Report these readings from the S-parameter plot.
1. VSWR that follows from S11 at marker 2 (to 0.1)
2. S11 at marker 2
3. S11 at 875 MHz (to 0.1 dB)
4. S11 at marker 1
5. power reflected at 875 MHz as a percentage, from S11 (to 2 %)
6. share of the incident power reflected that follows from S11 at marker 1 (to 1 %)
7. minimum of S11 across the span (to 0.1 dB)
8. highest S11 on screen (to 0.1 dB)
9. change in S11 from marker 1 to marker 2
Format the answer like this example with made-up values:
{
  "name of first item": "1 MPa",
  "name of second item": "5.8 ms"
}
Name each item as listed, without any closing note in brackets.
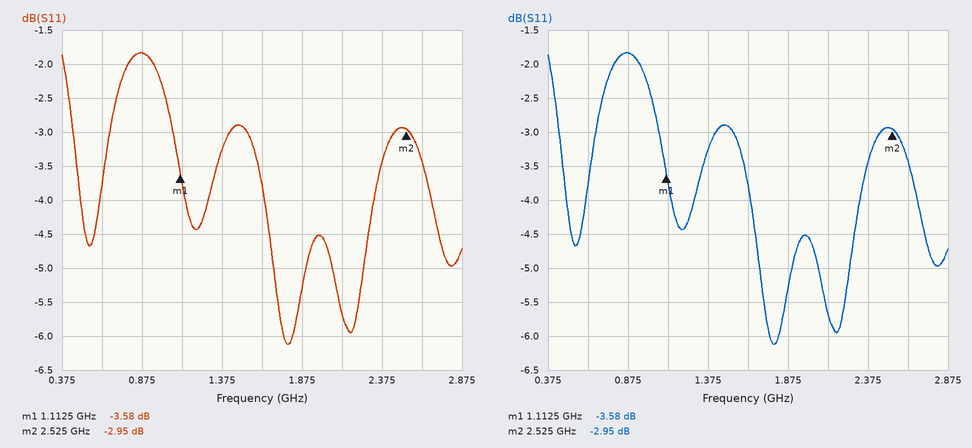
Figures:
{
  "VSWR that follows from S11 at marker 2": "5.9",
  "S11 at marker 2": "-2.95 dB",
  "S11 at 875 MHz": "-1.8 dB",
  "S11 at marker 1": "-3.58 dB",
  "power reflected at 875 MHz as a percentage, from S11": "66 %",
  "share of the incident power reflected that follows from S11 at marker 1": "44 %",
  "minimum of S11 across the span": "-6.1 dB",
  "highest S11 on screen": "-1.8 dB",
  "change in S11 from marker 1 to marker 2": "0.63 dB"
}
